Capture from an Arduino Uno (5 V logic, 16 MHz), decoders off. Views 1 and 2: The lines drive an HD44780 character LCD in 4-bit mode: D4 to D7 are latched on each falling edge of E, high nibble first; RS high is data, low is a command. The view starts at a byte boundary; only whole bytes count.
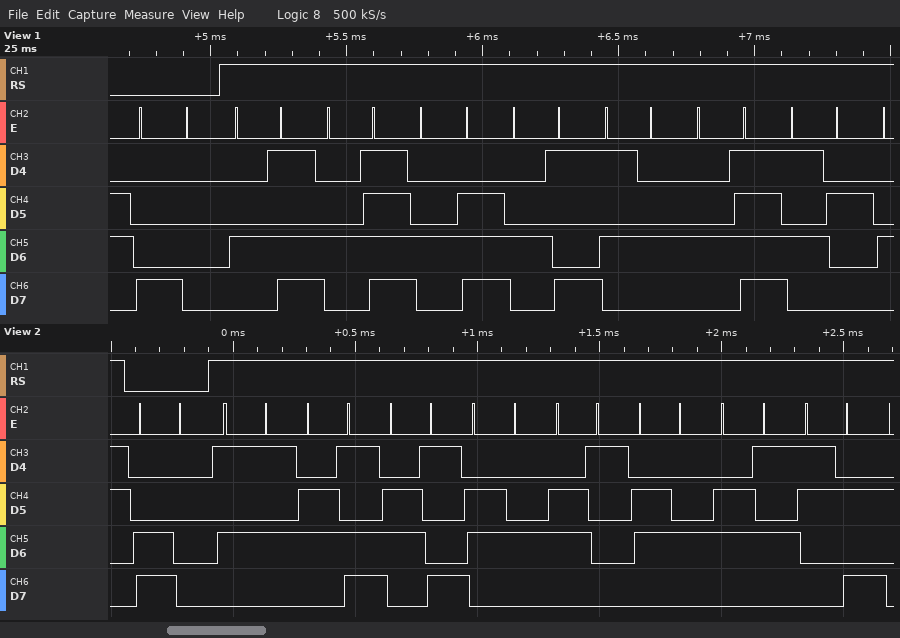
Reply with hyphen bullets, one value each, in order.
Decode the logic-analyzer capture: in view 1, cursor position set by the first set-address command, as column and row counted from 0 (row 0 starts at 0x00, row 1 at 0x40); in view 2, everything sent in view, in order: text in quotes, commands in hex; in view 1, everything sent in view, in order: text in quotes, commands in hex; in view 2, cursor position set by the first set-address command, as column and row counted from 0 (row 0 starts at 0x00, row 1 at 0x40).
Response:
- column 0, row 0
- 0xC0 "Umidade:"
- 0x80 "MONITOR"
- column 0, row 1
